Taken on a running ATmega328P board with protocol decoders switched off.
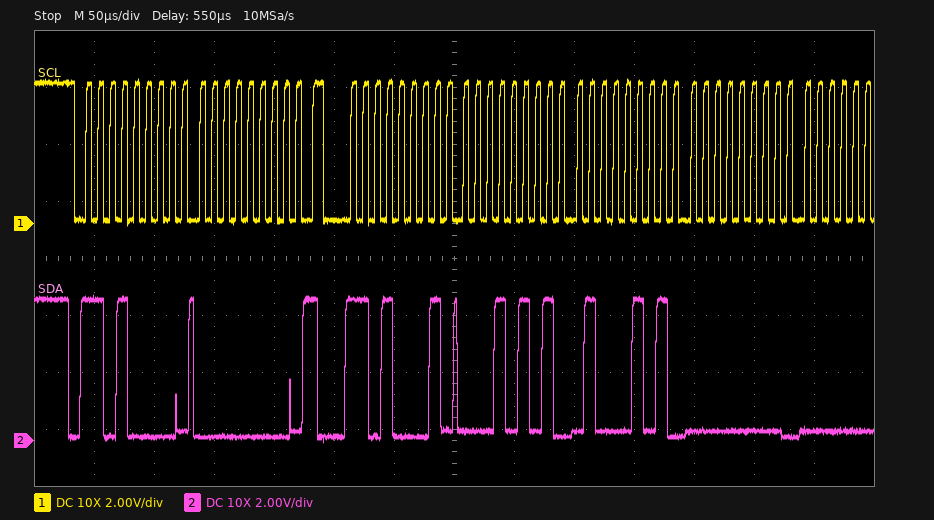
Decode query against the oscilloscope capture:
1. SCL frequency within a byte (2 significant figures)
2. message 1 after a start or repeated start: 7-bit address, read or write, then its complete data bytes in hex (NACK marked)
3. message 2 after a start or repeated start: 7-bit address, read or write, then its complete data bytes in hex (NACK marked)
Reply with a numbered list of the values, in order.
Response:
1. 100 kHz
2. 0x68 write: 00
3. 0x68 read: 15 45 00
